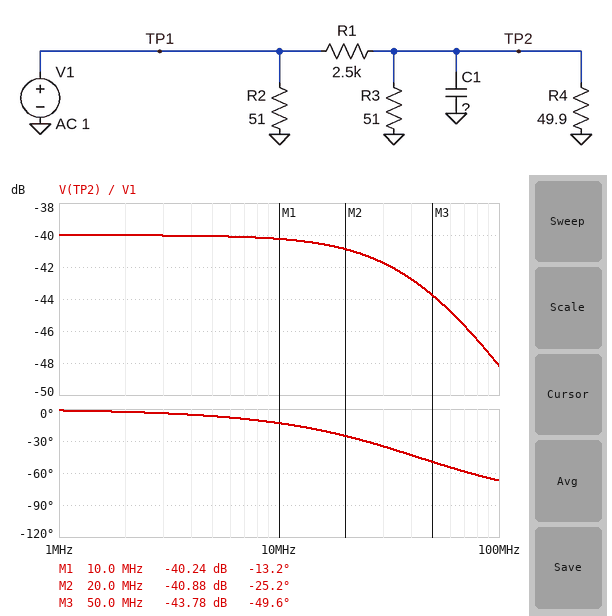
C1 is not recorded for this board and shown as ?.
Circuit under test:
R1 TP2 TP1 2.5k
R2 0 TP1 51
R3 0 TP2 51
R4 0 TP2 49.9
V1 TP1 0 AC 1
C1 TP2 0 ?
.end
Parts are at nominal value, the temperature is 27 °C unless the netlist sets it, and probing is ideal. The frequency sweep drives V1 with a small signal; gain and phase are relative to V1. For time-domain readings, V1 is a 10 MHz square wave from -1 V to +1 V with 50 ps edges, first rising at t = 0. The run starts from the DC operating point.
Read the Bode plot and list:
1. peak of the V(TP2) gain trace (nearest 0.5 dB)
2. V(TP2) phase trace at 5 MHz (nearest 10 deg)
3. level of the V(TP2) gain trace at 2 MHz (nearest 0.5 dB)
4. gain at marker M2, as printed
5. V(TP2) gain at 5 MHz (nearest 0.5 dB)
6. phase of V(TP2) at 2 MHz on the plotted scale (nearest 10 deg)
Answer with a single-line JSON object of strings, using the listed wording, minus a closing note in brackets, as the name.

{"peak of the V(TP2) gain trace": "-40.0 dB", "V(TP2) phase trace at 5 MHz": "-10 deg", "level of the V(TP2) gain trace at 2 MHz": "-40.0 dB", "gain at marker M2, as printed": "-40.88 dB", "V(TP2) gain at 5 MHz": "-40.0 dB", "phase of V(TP2) at 2 MHz on the plotted scale": "0 deg"}
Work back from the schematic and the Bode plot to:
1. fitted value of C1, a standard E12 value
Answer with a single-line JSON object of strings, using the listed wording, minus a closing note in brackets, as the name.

{"fitted value of C1, a standard E12 value": "150 pF"}
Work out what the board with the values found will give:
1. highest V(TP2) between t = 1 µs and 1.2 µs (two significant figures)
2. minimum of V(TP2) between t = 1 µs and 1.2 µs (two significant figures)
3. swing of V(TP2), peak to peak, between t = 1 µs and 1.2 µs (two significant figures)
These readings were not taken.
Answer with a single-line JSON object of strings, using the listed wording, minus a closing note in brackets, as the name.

{"highest V(TP2) between t = 1 µs and 1.2 µs": "10 mV", "minimum of V(TP2) between t = 1 µs and 1.2 µs": "-10 mV", "swing of V(TP2), peak to peak, between t = 1 µs and 1.2 µs": "20 mV"}
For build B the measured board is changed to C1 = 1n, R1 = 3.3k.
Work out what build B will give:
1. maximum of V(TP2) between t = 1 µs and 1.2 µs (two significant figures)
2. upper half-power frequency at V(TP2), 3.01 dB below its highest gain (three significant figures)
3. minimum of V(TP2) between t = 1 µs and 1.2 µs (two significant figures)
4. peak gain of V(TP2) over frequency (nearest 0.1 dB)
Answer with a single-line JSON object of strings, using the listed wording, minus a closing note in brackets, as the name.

{"maximum of V(TP2) between t = 1 µs and 1.2 µs": "5.8 mV", "upper half-power frequency at V(TP2), 3.01 dB below its highest gain": "6.36 MHz", "minimum of V(TP2) between t = 1 µs and 1.2 µs": "-5.8 mV", "peak gain of V(TP2) over frequency": "-42.4 dB"}
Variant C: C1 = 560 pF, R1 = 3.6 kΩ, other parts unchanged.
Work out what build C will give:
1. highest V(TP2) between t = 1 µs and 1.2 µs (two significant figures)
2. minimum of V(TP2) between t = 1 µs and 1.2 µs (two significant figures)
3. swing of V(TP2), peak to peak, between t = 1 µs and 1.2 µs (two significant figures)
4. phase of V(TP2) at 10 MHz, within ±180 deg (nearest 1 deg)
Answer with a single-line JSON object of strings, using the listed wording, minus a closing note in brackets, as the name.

{"highest V(TP2) between t = 1 µs and 1.2 µs": "6.6 mV", "minimum of V(TP2) between t = 1 µs and 1.2 µs": "-6.6 mV", "swing of V(TP2), peak to peak, between t = 1 µs and 1.2 µs": "13 mV", "phase of V(TP2) at 10 MHz, within ±180 deg": "-41 deg"}
